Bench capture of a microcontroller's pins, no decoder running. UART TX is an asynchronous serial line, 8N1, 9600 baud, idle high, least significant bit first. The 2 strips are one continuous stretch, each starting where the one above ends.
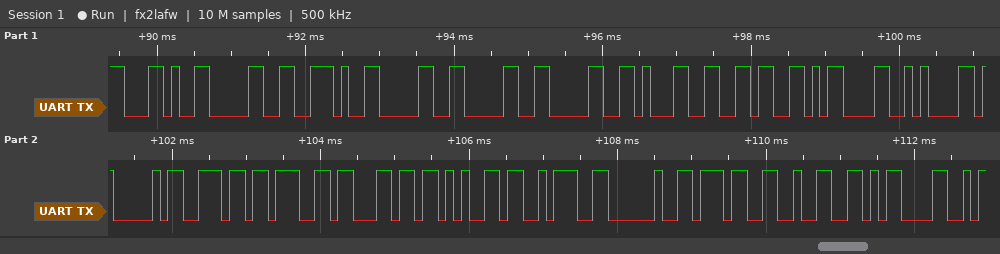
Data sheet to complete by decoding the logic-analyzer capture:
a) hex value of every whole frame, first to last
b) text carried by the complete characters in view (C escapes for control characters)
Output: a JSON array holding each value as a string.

["2C 30 2E 30 30 30 31 36 0D 0A 41 6E 67 6C 65 3A 20 37 32 0D", "\",0.00016\\r\\nAngle: 72\\r\""]
